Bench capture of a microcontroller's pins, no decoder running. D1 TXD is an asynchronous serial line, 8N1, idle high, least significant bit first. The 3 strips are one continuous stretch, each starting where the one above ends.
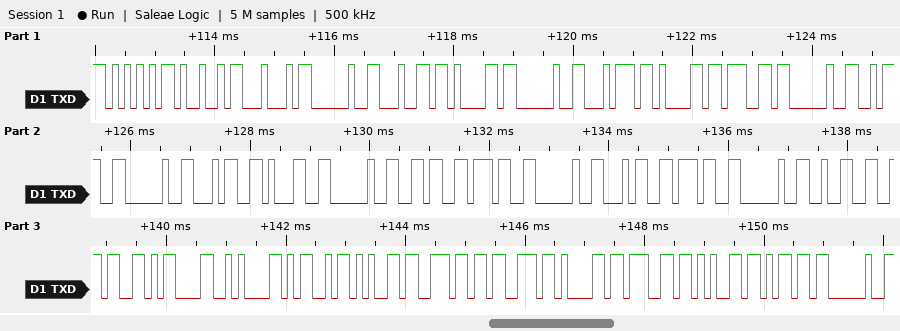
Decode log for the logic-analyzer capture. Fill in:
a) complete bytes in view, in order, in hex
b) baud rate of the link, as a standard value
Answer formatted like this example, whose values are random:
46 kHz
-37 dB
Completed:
0x55 0x49 0x44 0x20 0x64 0x61 0x20 0x74 0x61 0x67 0x20 0x3A 0x20 0x34 0x31 0x20 0x36 0x37 0x20 0x34 0x37 0x20 0x32 0x36 0x0D 0x0A 0x4D 0x65 0x6E 0x73 0x61 0x67 0x65 0x6D 0x20
9600 baud
